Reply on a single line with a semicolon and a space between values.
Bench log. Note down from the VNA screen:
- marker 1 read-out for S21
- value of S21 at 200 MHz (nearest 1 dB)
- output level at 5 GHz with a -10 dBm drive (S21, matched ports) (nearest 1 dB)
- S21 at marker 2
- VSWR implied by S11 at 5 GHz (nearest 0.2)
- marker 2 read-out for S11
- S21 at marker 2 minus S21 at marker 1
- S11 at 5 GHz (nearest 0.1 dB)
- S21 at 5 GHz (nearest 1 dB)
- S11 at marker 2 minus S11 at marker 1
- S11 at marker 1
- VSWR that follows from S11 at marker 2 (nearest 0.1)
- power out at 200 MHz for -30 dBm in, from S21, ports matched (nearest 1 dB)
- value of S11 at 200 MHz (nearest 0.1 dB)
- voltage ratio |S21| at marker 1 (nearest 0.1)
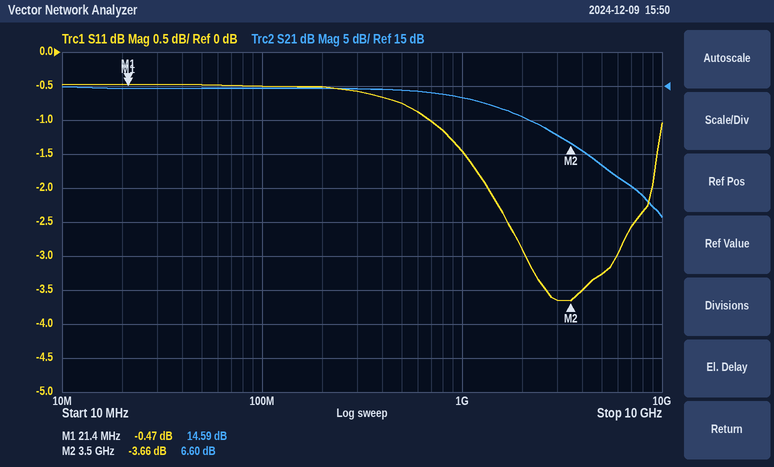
14.59 dB; 15 dB; -7 dBm; 6.60 dB; 5.4; -3.66 dB; -7.99 dB; -3.3 dB; 3 dB; -3.19 dB; -0.47 dB; 4.8; -15 dBm; -0.5 dB; 5.4
